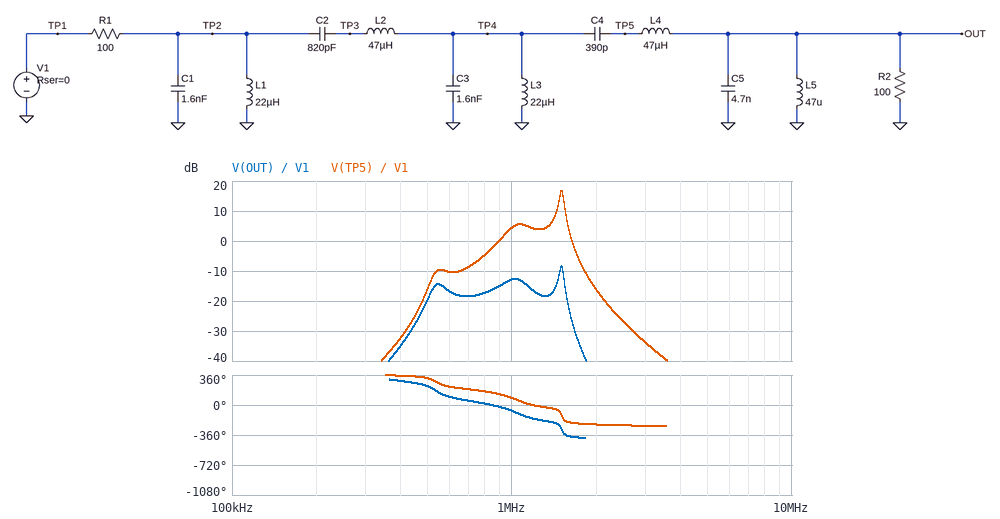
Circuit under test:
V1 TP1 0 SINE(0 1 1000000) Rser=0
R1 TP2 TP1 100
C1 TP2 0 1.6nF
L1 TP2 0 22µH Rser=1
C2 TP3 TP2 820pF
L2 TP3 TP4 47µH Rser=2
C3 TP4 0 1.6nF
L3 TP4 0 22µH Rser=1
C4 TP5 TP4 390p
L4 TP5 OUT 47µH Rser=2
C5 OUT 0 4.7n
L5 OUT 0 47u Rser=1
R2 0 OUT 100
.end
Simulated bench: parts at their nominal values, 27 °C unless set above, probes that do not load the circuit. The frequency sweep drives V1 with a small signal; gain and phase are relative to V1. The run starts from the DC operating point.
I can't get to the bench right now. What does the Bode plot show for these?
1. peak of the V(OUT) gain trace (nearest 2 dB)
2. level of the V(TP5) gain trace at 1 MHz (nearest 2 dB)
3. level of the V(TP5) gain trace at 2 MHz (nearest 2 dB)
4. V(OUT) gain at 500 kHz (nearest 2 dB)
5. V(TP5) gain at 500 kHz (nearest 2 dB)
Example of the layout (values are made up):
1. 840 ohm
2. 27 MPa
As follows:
1. -8 dB
2. 4 dB
3. -16 dB
4. -20 dB
5. -16 dB
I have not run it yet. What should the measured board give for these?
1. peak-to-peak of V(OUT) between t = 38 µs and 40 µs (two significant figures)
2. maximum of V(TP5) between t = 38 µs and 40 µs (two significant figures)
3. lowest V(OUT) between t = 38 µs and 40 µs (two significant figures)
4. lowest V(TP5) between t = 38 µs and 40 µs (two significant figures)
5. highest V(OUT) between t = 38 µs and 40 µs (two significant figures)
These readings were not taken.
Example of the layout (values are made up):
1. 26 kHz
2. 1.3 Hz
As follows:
1. 460 mV
2. 1.7 V
3. -230 mV
4. -1.7 V
5. 230 mV
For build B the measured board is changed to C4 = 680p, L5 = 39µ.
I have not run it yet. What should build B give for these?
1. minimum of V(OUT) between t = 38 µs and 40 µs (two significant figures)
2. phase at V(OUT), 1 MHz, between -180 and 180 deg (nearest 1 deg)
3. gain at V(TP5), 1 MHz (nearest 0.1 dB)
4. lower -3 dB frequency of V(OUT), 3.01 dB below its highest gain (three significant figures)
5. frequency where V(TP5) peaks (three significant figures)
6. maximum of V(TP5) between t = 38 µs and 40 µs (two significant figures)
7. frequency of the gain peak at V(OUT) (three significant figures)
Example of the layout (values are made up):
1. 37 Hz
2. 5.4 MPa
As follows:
1. -250 mV
2. -130 deg
3. 5.0 dB
4. 496 kHz
5. 1.39 MHz
6. 1.8 V
7. 527 kHz
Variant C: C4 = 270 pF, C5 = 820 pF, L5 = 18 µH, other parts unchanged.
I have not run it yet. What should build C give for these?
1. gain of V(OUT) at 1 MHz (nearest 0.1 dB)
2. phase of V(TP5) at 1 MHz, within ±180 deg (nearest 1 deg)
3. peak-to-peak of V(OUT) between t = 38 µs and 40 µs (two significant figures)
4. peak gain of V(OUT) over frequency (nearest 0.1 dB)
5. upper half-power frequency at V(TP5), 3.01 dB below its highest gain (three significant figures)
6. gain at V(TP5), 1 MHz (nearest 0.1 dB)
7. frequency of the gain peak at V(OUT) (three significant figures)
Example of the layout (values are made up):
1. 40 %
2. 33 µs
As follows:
1. -9.3 dB
2. 84 deg
3. 690 mV
4. -7.7 dB
5. 1.35 MHz
6. 2.0 dB
7. 1.11 MHz
